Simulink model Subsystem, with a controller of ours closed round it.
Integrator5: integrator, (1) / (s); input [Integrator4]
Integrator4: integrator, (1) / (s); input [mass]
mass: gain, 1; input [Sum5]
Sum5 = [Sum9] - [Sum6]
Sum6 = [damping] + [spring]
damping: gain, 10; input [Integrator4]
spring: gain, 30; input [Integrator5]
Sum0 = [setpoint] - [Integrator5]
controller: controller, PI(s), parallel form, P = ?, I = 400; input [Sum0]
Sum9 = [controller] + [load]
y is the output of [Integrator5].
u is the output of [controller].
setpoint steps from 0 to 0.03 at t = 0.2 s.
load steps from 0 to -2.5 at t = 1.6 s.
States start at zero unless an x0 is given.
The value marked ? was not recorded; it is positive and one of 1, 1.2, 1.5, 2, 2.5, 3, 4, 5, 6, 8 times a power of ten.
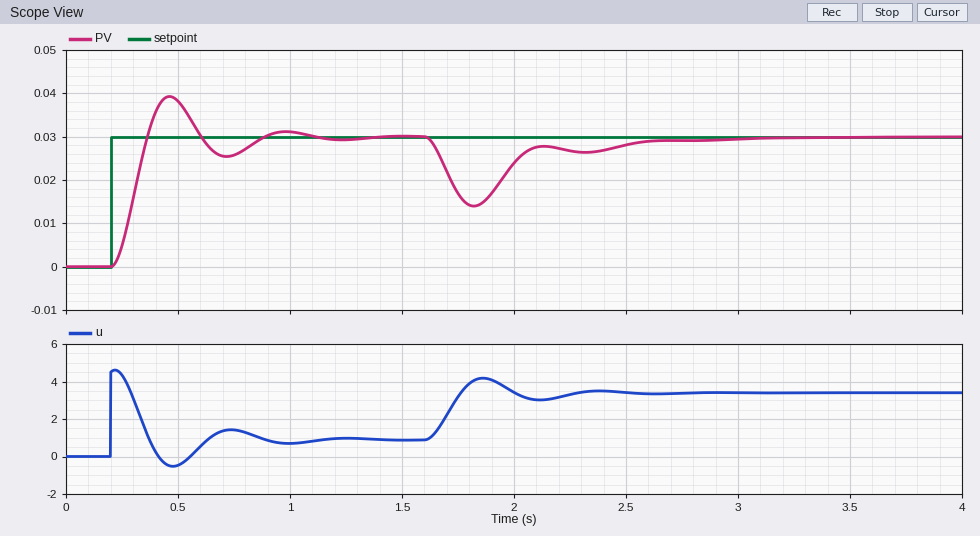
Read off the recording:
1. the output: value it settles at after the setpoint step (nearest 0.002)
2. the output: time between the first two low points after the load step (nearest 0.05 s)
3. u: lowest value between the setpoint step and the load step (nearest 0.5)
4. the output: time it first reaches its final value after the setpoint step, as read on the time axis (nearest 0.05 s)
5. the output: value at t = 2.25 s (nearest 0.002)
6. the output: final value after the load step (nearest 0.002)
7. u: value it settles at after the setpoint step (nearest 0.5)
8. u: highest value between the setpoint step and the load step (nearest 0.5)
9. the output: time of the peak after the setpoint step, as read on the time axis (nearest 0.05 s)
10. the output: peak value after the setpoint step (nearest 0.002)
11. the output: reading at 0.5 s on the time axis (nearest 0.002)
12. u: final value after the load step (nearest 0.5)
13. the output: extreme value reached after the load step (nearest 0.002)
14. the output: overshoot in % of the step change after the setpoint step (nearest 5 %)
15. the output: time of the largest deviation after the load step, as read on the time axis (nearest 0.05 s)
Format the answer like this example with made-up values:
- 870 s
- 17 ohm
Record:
- 0.030
- 0.50 s
- -0.5
- 0.35 s
- 0.026
- 0.030
- 1.0
- 4.5
- 0.45 s
- 0.040
- 0.038
- 3.5
- 0.014
- 30 %
- 1.80 s
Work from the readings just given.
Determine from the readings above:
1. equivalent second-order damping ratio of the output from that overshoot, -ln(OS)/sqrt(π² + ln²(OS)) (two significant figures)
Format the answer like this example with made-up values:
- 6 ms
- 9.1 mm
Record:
- 0.36
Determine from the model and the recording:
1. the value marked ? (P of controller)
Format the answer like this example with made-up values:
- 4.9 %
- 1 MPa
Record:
- 150
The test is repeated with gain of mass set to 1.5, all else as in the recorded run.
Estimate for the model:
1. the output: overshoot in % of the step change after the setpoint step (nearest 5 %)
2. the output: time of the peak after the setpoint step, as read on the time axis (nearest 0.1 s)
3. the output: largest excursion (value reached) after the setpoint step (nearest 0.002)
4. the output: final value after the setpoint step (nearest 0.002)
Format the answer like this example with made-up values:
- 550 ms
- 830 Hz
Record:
- 20 %
- 0.4 s
- 0.036
- 0.030
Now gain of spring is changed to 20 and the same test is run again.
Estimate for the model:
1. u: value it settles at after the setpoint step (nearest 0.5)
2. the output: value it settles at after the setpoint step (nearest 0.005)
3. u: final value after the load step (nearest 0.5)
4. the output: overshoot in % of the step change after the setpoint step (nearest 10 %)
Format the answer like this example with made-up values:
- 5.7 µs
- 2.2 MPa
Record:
- 0.5
- 0.030
- 3.0
- 40 %
